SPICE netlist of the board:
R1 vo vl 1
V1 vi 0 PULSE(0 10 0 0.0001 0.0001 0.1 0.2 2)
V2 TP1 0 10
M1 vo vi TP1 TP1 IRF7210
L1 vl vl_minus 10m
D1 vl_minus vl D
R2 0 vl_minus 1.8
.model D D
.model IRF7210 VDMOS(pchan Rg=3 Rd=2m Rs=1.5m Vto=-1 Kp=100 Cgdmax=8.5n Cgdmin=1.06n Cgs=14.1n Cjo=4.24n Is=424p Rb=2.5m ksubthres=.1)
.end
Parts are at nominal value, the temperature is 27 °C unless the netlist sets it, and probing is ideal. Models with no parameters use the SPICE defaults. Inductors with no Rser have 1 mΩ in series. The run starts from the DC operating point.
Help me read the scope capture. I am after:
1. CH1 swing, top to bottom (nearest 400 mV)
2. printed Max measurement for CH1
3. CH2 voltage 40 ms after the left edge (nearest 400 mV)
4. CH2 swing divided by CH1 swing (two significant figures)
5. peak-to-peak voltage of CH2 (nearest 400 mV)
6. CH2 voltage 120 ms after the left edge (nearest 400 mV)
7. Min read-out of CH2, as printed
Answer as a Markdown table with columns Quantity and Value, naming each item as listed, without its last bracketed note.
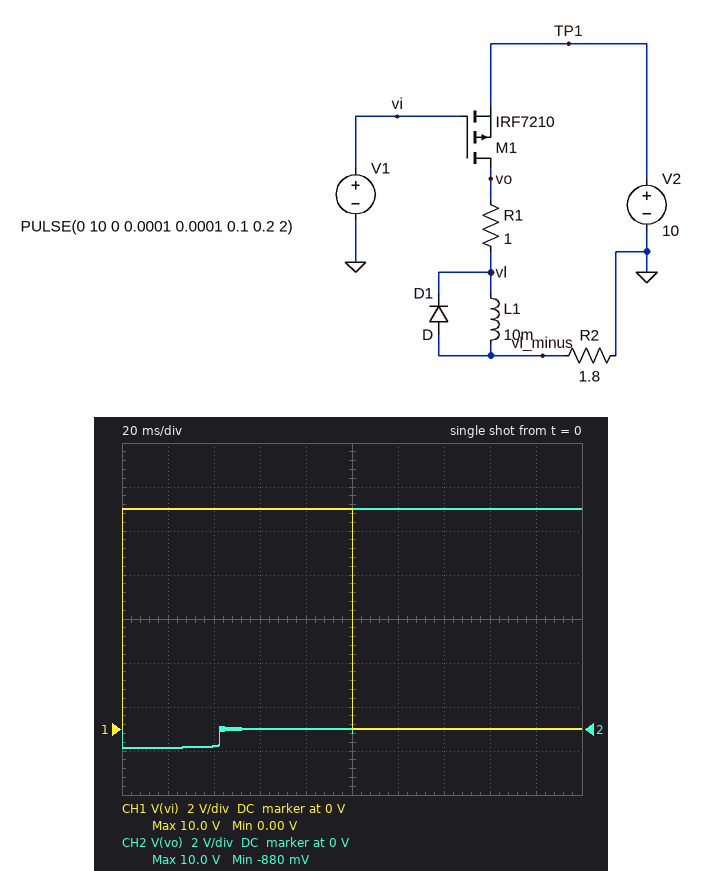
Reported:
| Quantity | Value |
|---|---|
| CH1 swing, top to bottom | 10.0 V |
| printed Max measurement for CH1 | 10.0 V |
| CH2 voltage 40 ms after the left edge | -800 mV |
| CH2 swing divided by CH1 swing | 1.1 |
| peak-to-peak voltage of CH2 | 10.8 V |
| CH2 voltage 120 ms after the left edge | 10.0 V |
| Min read-out of CH2, as printed | -880 mV |
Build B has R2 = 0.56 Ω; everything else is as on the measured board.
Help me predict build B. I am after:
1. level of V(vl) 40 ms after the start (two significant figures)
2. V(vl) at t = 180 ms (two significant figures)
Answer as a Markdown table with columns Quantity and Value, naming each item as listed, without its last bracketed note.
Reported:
| Quantity | Value |
|---|---|
| level of V(vl) 40 ms after the start | -860 mV |
| V(vl) at t = 180 ms | 3.6 V |
